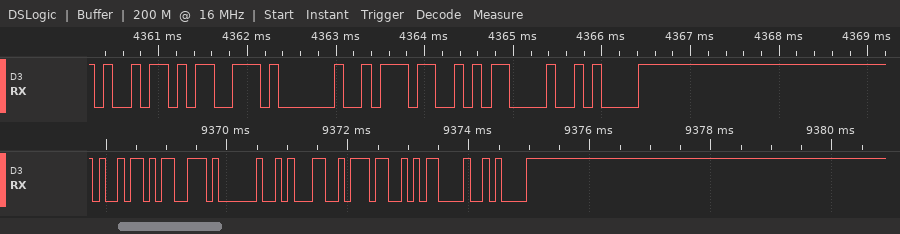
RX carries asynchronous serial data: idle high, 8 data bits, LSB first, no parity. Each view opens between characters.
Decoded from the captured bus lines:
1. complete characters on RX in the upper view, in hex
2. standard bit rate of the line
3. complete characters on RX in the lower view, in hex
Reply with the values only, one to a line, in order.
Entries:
69, 73, 20, 37, 0D, 0A
9600 baud
69, 73, 20, 31, 37, 0D, 0A
